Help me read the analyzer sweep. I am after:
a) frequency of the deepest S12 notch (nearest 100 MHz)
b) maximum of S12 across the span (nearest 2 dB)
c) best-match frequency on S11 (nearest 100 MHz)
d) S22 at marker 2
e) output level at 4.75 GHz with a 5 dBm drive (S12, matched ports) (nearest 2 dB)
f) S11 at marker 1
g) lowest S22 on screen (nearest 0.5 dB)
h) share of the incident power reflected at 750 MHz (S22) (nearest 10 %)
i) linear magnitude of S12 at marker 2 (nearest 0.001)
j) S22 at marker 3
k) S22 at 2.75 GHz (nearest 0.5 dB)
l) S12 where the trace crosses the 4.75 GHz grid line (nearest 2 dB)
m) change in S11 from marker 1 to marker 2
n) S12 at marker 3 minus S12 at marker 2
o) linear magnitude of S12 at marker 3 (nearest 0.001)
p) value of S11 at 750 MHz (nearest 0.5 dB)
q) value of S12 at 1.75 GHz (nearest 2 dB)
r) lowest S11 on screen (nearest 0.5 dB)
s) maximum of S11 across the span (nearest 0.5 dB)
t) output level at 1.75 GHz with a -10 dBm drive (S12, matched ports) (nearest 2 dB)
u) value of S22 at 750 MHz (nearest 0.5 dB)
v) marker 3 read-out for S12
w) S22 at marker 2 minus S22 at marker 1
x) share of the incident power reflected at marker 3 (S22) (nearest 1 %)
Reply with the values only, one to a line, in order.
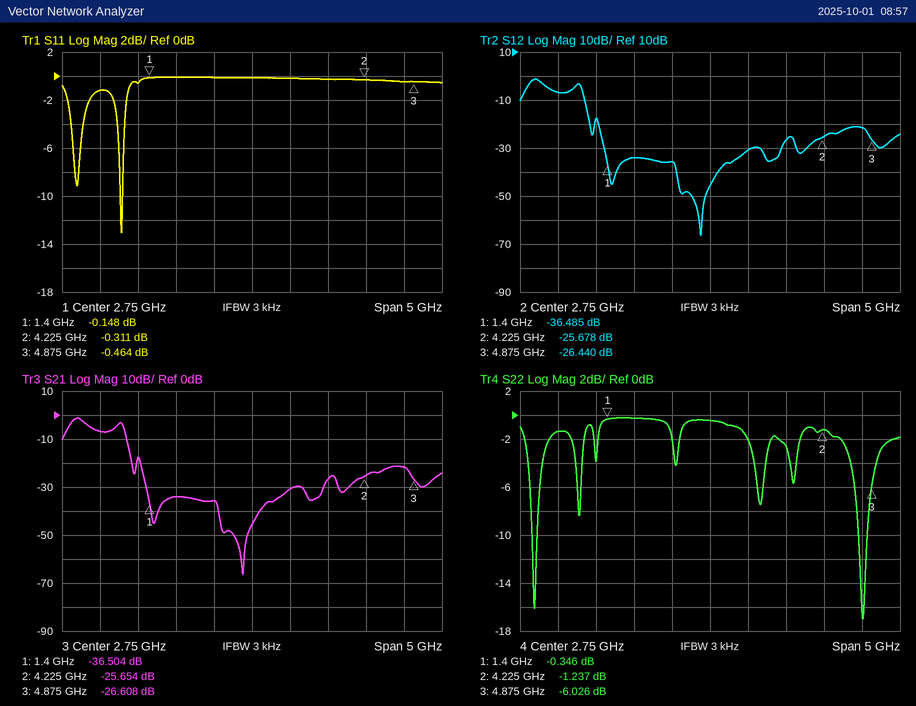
2.6 GHz
-2 dB
1.0 GHz
-1.237 dB
-16 dBm
-0.148 dB
-17.0 dB
70 %
0.052
-6.026 dB
-0.5 dB
-22 dB
-0.163 dB
-0.762 dB
0.048
-1.0 dB
-34 dB
-13.0 dB
0.0 dB
-44 dBm
-1.5 dB
-26.440 dB
-0.891 dB
25 %
